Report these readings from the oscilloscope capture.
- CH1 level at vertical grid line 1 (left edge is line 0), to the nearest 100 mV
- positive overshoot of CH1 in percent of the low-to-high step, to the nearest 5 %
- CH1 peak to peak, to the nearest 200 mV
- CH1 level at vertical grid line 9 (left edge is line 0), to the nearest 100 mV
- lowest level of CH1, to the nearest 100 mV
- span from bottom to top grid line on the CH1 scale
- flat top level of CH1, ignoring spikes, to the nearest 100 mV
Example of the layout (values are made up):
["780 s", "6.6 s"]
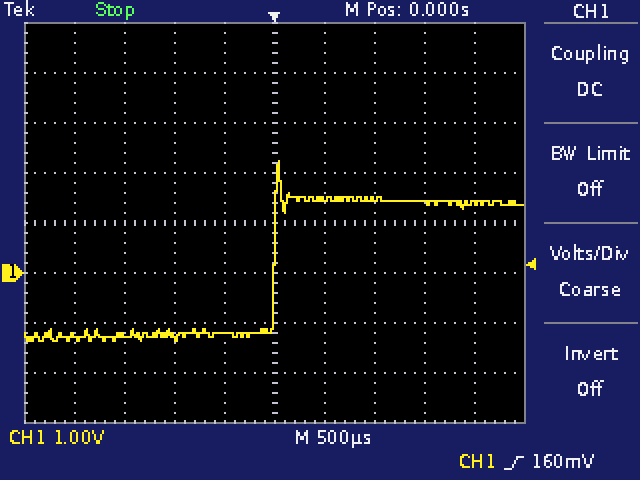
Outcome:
["-1.3 V", "30 %", "3.6 V", "1.4 V", "-1.4 V", "8 V", "1.4 V"]
